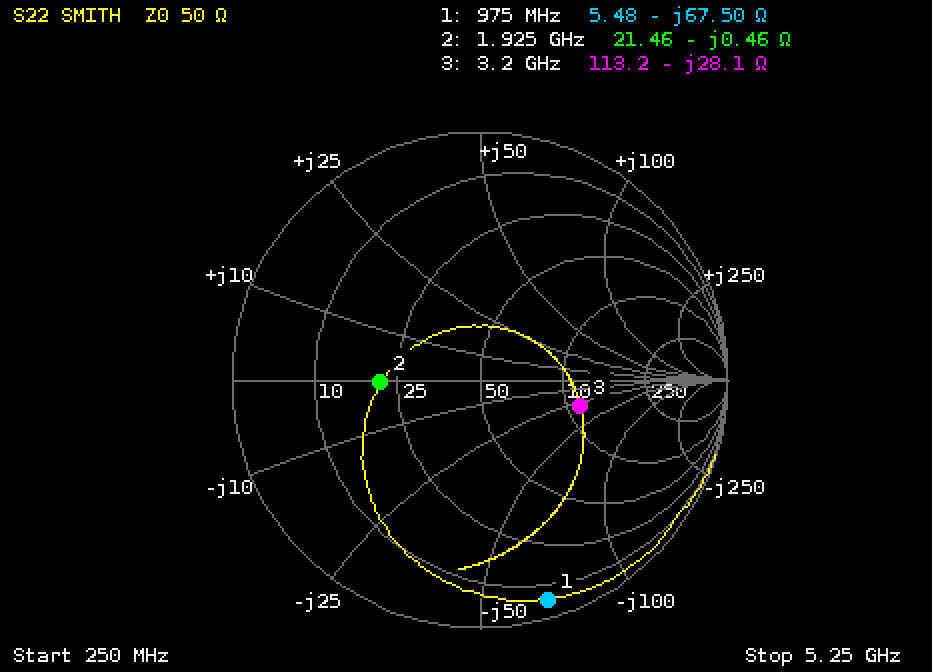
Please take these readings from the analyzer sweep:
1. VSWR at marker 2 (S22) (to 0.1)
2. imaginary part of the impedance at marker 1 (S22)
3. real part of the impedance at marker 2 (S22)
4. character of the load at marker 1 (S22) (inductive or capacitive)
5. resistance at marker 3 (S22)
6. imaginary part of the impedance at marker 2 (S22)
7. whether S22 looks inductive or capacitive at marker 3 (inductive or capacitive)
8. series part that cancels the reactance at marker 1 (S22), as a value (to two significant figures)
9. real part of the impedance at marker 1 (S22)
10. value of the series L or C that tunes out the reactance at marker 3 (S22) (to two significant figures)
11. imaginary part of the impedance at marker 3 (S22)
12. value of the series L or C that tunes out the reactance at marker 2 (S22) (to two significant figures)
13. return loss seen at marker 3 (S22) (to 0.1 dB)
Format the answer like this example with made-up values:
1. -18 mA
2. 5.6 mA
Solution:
1. 2.3
2. -67.50 Ω
3. 21.46 Ω
4. capacitive
5. 113.2 Ω
6. -0.46 Ω
7. capacitive
8. 11 nH
9. 5.48 Ω
10. 1.4 nH
11. -28.1 Ω
12. 38 pH
13. 7.6 dB
